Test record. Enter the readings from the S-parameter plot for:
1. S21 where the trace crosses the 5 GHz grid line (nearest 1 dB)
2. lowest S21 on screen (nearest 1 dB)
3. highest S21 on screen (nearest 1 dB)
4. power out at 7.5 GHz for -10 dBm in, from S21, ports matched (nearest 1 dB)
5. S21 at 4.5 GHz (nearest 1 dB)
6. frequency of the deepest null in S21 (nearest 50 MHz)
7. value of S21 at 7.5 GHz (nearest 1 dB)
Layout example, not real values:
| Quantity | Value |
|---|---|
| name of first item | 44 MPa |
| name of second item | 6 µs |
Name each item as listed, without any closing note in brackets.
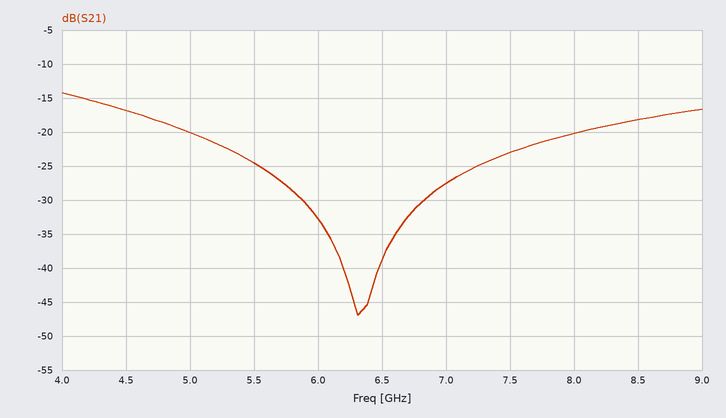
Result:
| Quantity | Value |
|---|---|
| S21 where the trace crosses the 5 GHz grid line | -20 dB |
| lowest S21 on screen | -47 dB |
| highest S21 on screen | -14 dB |
| power out at 7.5 GHz for -10 dBm in, from S21, ports matched | -33 dBm |
| S21 at 4.5 GHz | -17 dB |
| frequency of the deepest null in S21 | 6.30 GHz |
| value of S21 at 7.5 GHz | -23 dB |
